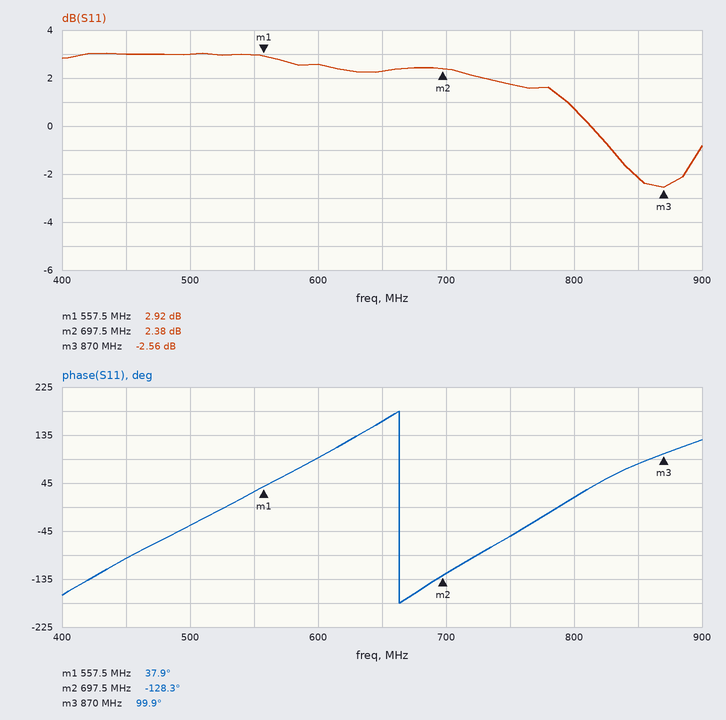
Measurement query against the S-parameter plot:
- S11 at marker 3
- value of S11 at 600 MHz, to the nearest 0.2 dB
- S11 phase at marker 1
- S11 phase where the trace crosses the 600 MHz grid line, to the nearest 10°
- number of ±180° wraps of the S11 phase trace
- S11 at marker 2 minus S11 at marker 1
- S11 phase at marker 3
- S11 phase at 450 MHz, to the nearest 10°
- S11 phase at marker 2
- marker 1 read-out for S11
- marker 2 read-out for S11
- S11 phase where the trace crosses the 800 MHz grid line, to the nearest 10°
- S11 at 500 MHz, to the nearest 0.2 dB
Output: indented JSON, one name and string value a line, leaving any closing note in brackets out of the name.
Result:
{
  "S11 at marker 3": "-2.56 dB",
  "value of S11 at 600 MHz, to the nearest 0.2 dB": "2.6 dB",
  "S11 phase at marker 1": "37.9°",
  "S11 phase where the trace crosses the 600 MHz grid line, to the nearest 10°": "90°",
  "number of ±180° wraps of the S11 phase trace": "1",
  "S11 at marker 2 minus S11 at marker 1": "-0.54 dB",
  "S11 phase at marker 3": "99.9°",
  "S11 phase at 450 MHz, to the nearest 10°": "-100°",
  "S11 phase at marker 2": "-128.3°",
  "marker 1 read-out for S11": "2.92 dB",
  "marker 2 read-out for S11": "2.38 dB",
  "S11 phase where the trace crosses the 800 MHz grid line, to the nearest 10°": "20°",
  "S11 at 500 MHz, to the nearest 0.2 dB": "3.0 dB"
}
